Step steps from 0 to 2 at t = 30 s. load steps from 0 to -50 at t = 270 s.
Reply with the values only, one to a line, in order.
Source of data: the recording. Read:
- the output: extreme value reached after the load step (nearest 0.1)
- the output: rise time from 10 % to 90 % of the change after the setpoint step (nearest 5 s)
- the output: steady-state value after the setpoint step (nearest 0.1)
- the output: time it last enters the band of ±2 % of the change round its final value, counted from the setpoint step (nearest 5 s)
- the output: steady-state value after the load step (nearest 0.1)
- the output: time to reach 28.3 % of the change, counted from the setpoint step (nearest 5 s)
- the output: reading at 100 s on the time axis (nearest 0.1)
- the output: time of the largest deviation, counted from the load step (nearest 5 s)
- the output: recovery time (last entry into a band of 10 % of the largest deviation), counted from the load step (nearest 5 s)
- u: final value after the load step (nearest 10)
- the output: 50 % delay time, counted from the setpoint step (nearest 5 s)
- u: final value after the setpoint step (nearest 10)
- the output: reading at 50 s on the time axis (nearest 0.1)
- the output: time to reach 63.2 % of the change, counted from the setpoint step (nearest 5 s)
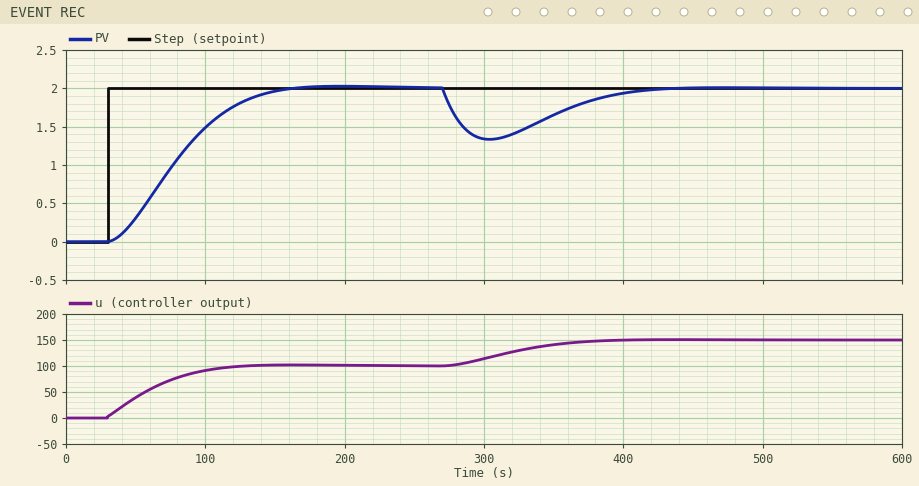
1.3
80 s
2.0
120 s
2.0
30 s
1.5
35 s
130 s
150
45 s
100
0.3
60 s
